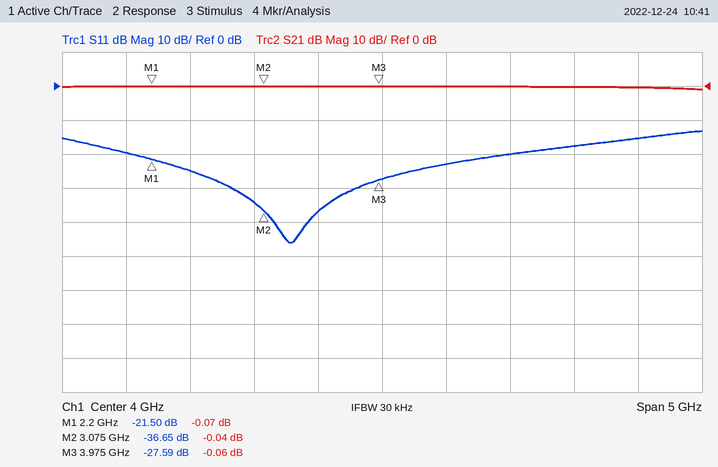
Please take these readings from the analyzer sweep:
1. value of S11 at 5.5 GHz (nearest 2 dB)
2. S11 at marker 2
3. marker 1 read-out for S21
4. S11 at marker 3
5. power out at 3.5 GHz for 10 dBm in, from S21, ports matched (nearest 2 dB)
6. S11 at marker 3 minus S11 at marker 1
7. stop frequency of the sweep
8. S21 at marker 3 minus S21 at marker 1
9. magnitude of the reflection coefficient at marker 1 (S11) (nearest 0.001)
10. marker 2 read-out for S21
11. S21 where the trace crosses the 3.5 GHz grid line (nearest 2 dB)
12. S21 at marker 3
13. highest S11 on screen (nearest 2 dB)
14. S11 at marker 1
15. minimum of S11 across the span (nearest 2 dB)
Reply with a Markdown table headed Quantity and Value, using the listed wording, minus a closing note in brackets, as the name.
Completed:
| Quantity | Value |
|---|---|
| value of S11 at 5.5 GHz | -18 dB |
| S11 at marker 2 | -36.65 dB |
| marker 1 read-out for S21 | -0.07 dB |
| S11 at marker 3 | -27.59 dB |
| power out at 3.5 GHz for 10 dBm in, from S21, ports matched | 10 dBm |
| S11 at marker 3 minus S11 at marker 1 | -6.09 dB |
| stop frequency of the sweep | 6.5 GHz |
| S21 at marker 3 minus S21 at marker 1 | 0.01 dB |
| magnitude of the reflection coefficient at marker 1 (S11) | 0.084 |
| marker 2 read-out for S21 | -0.04 dB |
| S21 where the trace crosses the 3.5 GHz grid line | 0 dB |
| S21 at marker 3 | -0.06 dB |
| highest S11 on screen | -14 dB |
| S11 at marker 1 | -21.50 dB |
| minimum of S11 across the span | -46 dB |
